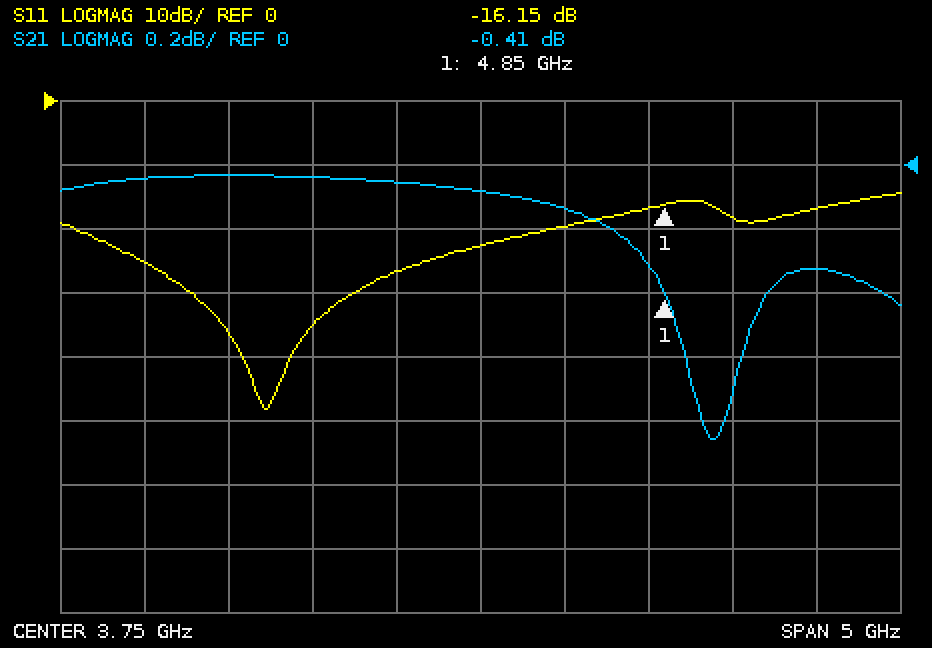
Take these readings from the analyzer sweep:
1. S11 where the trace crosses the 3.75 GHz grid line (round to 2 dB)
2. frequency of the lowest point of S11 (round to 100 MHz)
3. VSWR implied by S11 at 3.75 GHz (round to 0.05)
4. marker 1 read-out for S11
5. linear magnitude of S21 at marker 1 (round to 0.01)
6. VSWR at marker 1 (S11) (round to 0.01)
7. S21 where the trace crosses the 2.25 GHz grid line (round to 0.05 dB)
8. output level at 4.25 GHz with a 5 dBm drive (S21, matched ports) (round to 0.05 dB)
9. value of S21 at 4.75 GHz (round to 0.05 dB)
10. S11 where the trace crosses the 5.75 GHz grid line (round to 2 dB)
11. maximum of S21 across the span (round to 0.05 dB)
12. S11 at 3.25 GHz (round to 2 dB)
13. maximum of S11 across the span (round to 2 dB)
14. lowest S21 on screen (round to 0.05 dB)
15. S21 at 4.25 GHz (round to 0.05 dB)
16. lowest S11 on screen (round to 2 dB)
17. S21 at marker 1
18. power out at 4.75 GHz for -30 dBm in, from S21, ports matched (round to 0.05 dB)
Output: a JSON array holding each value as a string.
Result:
["-22 dB", "2.5 GHz", "1.15", "-16.15 dB", "0.95", "1.37", "-0.05 dB", "4.85 dBm", "-0.30 dB", "-16 dB", "-0.05 dB", "-26 dB", "-14 dB", "-0.85 dB", "-0.15 dB", "-48 dB", "-0.41 dB", "-30.30 dBm"]
